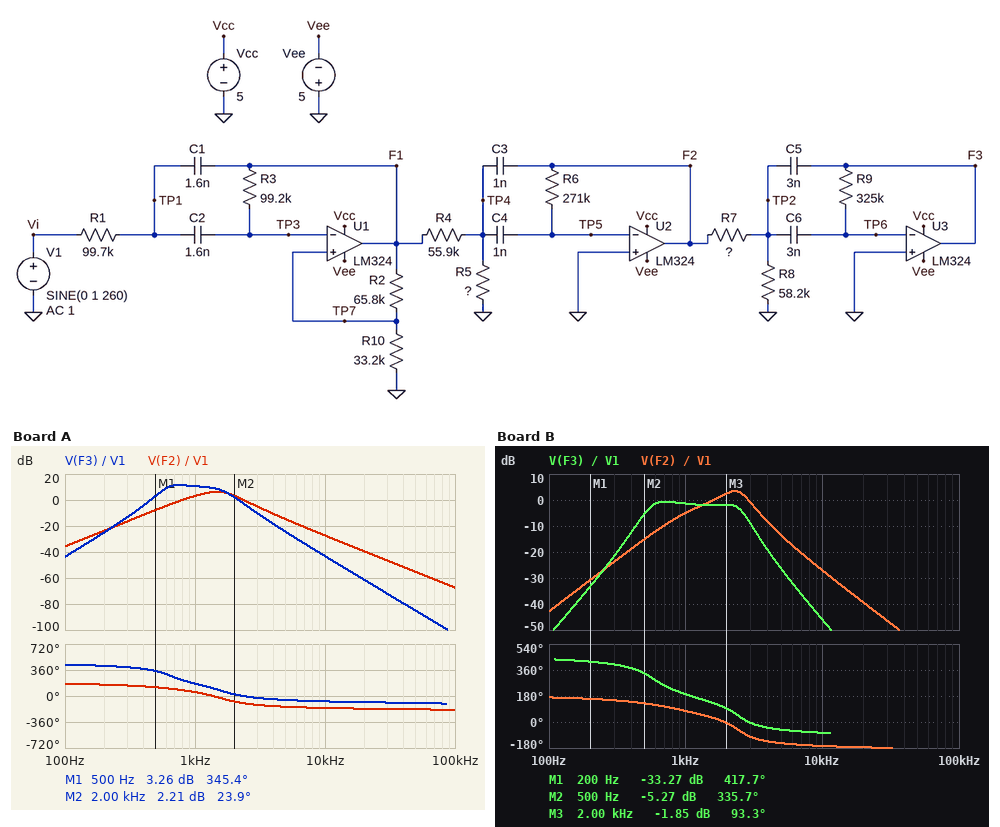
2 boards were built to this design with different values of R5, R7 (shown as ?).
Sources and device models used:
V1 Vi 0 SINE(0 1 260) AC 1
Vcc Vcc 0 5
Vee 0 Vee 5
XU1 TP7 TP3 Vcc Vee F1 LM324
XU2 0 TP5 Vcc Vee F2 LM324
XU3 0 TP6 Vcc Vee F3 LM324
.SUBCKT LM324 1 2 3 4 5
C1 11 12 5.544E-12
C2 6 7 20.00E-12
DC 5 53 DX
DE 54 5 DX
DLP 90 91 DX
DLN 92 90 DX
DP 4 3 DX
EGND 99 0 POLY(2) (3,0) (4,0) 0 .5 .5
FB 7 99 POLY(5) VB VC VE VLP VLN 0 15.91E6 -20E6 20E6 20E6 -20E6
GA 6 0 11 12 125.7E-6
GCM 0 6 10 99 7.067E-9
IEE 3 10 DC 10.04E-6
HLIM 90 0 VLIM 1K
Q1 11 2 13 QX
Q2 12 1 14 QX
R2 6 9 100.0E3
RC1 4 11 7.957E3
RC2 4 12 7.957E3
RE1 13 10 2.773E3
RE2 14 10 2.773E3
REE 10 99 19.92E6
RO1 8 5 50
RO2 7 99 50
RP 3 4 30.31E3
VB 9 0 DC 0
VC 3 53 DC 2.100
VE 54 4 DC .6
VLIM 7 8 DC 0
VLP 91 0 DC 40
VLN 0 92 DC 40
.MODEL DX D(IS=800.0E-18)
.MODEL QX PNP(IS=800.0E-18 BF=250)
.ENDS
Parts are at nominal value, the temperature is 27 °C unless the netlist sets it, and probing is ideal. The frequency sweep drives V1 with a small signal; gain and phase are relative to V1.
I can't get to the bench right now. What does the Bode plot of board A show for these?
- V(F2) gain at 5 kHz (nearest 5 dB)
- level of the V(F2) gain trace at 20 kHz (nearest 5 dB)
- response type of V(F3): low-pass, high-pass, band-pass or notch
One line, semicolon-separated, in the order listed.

-15 dB; -40 dB; band-pass
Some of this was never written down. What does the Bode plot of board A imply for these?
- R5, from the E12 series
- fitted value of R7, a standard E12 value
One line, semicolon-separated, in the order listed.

100 kΩ; 33 kΩ
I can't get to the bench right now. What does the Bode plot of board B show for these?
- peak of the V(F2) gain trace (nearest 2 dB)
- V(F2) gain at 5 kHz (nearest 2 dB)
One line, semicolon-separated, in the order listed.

4 dB; -14 dB
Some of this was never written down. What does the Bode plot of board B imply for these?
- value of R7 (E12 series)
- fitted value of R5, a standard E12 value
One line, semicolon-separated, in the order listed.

47 kΩ; 22 kΩ
